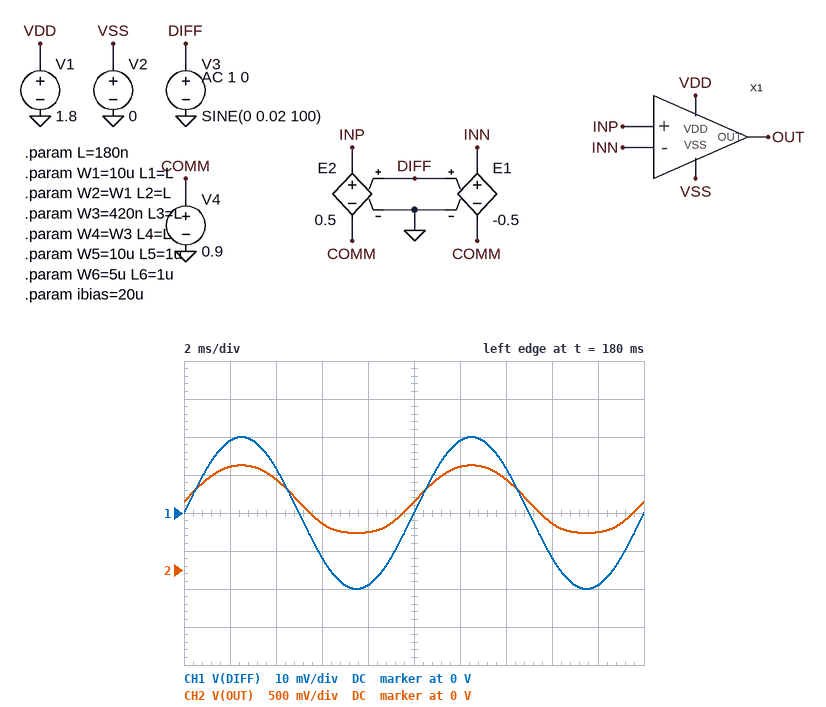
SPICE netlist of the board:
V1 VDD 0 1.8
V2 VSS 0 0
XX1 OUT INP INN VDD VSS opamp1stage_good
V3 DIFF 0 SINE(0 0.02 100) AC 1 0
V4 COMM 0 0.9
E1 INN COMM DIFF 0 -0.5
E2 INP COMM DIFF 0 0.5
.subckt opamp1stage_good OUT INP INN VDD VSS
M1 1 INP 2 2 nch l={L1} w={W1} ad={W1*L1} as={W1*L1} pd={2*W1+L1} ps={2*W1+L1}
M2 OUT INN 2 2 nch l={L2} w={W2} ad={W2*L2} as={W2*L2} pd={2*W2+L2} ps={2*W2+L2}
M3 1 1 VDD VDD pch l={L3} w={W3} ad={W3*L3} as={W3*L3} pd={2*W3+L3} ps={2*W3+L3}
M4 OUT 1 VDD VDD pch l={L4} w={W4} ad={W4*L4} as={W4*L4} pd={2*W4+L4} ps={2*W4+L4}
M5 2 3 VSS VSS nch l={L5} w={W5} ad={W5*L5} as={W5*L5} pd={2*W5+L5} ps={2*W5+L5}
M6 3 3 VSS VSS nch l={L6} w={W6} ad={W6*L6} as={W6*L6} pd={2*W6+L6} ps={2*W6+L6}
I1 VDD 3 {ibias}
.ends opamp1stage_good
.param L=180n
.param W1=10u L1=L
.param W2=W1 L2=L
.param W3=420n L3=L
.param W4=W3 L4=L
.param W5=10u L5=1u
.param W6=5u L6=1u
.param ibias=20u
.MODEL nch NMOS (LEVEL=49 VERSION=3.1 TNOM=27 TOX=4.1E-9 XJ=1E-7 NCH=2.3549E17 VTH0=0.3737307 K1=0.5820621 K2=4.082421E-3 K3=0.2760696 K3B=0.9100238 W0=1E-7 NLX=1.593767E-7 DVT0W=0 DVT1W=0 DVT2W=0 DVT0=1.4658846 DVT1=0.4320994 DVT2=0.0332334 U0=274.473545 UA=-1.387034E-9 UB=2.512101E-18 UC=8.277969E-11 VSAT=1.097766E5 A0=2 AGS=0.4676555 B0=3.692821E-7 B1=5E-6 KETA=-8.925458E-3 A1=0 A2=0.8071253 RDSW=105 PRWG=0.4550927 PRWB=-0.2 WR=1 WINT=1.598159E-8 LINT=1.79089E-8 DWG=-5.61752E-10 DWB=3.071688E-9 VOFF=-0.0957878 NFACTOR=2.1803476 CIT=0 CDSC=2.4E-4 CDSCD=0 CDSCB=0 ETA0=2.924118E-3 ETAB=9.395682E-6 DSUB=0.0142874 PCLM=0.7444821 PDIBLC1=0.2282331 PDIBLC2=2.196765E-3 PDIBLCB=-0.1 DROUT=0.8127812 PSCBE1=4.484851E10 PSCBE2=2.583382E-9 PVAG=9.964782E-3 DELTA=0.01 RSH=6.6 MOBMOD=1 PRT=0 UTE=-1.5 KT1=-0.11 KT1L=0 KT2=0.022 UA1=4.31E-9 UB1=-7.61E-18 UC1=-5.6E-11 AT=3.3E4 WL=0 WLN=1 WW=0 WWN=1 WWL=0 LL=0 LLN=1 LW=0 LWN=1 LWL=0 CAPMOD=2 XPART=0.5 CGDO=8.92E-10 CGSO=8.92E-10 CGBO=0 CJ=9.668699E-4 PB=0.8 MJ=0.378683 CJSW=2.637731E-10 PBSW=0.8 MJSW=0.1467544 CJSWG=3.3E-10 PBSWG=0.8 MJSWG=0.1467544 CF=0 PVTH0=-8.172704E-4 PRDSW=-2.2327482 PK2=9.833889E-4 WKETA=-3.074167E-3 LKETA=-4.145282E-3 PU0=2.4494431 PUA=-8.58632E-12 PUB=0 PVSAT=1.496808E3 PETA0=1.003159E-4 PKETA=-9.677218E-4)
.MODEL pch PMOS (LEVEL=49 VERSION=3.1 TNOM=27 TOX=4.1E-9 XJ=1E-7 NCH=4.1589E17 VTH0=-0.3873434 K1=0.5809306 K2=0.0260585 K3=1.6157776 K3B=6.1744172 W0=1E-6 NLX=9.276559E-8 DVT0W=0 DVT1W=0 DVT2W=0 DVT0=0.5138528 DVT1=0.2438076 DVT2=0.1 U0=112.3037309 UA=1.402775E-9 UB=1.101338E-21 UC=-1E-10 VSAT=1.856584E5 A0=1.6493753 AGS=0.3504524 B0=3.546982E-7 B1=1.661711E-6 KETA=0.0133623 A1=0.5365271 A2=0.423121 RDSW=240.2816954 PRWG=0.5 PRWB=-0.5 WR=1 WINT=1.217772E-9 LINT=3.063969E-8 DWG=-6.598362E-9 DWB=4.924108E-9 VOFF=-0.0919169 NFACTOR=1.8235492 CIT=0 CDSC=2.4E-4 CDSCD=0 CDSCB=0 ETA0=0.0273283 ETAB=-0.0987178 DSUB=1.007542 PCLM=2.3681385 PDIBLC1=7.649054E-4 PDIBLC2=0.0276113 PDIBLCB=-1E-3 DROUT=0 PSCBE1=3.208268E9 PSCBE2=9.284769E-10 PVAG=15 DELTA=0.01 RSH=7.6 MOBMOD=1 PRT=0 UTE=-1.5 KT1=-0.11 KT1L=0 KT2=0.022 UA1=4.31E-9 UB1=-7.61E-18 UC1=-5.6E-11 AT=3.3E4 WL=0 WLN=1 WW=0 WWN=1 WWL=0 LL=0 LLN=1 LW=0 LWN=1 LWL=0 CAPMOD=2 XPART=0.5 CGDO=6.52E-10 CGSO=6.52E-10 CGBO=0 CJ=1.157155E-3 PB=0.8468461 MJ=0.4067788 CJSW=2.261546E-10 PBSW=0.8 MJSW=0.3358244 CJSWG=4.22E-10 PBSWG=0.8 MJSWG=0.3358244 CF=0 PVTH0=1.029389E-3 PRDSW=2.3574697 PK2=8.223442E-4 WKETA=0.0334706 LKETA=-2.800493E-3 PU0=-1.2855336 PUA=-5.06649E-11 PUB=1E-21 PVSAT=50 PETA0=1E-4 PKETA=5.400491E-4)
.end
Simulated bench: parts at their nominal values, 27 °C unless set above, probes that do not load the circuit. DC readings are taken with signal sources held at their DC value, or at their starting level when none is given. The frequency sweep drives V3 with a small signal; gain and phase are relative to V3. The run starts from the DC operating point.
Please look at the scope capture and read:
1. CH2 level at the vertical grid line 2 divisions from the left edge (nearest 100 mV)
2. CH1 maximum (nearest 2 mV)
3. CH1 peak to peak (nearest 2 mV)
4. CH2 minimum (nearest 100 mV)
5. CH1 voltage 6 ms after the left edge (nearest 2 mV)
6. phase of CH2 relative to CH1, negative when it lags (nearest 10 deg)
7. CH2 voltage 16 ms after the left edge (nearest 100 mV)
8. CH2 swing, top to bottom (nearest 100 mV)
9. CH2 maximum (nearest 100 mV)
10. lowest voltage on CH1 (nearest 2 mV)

1.2 V
20 mV
40 mV
500 mV
-12 mV
0 deg
600 mV
900 mV
1.4 V
-20 mV
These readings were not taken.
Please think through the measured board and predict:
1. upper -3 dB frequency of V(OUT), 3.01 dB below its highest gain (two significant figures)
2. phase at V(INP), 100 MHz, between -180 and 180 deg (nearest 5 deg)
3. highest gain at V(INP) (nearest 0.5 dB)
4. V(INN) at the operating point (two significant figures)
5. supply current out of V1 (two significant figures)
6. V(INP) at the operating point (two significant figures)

150 MHz
0 deg
-6.0 dB
900 mV
59 µA
900 mV
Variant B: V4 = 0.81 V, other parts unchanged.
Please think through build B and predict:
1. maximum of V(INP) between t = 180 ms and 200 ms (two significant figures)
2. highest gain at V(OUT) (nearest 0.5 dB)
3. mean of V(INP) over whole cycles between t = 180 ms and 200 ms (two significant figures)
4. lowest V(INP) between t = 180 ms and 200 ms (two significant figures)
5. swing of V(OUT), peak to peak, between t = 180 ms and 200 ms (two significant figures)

820 mV
28.5 dB
810 mV
800 mV
950 mV
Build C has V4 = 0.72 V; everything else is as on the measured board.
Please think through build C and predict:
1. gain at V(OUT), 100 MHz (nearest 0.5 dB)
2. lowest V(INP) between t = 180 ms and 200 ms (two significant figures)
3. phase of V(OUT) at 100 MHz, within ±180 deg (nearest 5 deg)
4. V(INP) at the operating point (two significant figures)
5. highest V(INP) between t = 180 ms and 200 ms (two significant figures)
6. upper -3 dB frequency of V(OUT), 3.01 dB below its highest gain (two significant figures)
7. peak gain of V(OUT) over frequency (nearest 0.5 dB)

27.0 dB
710 mV
-40 deg
720 mV
730 mV
140 MHz
28.5 dB
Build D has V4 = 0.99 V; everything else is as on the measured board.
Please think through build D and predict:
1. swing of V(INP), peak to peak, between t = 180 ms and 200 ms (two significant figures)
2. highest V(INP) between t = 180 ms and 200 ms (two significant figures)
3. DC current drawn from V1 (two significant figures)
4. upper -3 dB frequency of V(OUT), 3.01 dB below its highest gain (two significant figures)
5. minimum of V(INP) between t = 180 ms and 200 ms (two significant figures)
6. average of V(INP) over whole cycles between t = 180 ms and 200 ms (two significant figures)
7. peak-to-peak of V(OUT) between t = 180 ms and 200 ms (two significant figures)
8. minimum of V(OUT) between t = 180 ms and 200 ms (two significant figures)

20 mV
1.0 V
60 µA
160 MHz
980 mV
990 mV
810 mV
560 mV
